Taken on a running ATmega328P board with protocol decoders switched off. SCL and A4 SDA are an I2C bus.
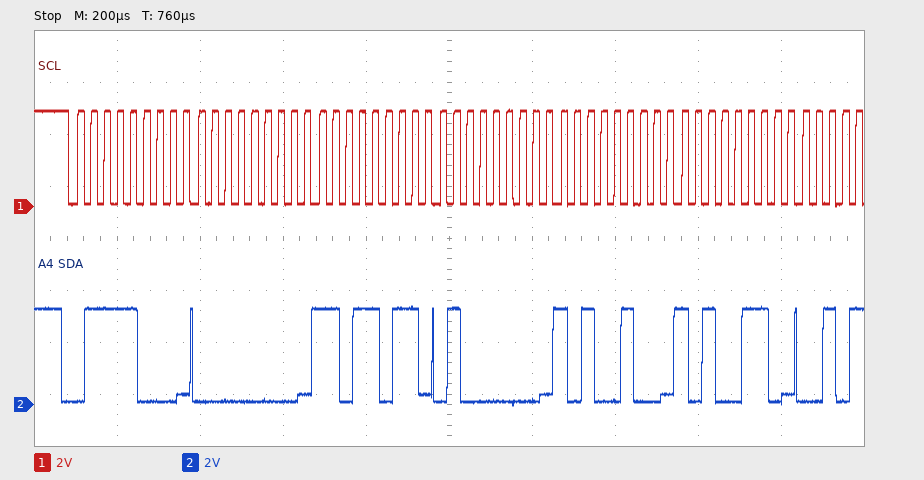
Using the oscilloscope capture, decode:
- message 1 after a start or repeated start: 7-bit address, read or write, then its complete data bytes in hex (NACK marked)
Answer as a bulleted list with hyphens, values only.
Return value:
- 0x3C write: 00 DB 40 A4 A6
